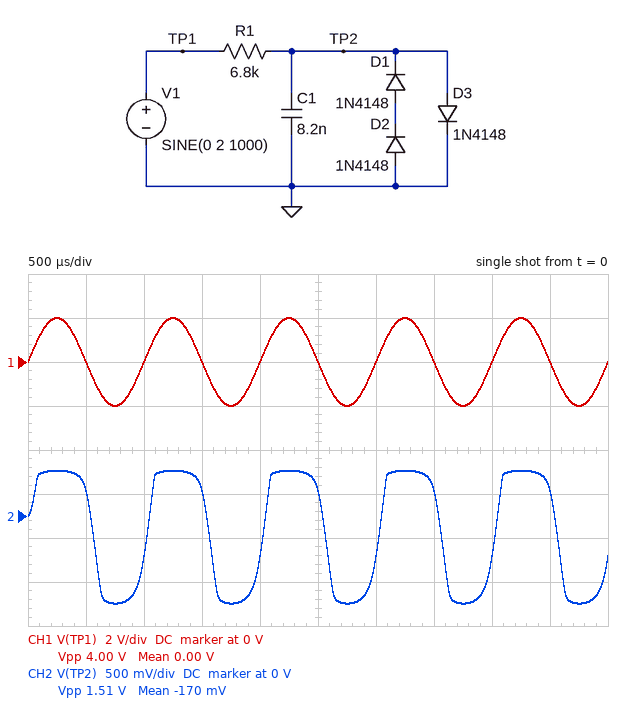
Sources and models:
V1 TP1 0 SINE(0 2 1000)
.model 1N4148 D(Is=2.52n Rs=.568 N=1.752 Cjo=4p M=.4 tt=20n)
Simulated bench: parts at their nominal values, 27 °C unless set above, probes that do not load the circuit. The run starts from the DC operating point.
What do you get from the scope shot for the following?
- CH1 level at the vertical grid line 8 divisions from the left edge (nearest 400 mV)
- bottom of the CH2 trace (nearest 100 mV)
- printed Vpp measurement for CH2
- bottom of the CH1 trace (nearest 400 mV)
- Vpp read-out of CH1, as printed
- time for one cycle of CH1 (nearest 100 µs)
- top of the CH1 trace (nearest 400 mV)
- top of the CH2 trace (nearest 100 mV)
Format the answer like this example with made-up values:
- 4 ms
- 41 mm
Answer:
- 0 V
- -1.0 V
- 1.51 V
- -2.0 V
- 4.00 V
- 1.0 ms
- 2.0 V
- 500 mV
